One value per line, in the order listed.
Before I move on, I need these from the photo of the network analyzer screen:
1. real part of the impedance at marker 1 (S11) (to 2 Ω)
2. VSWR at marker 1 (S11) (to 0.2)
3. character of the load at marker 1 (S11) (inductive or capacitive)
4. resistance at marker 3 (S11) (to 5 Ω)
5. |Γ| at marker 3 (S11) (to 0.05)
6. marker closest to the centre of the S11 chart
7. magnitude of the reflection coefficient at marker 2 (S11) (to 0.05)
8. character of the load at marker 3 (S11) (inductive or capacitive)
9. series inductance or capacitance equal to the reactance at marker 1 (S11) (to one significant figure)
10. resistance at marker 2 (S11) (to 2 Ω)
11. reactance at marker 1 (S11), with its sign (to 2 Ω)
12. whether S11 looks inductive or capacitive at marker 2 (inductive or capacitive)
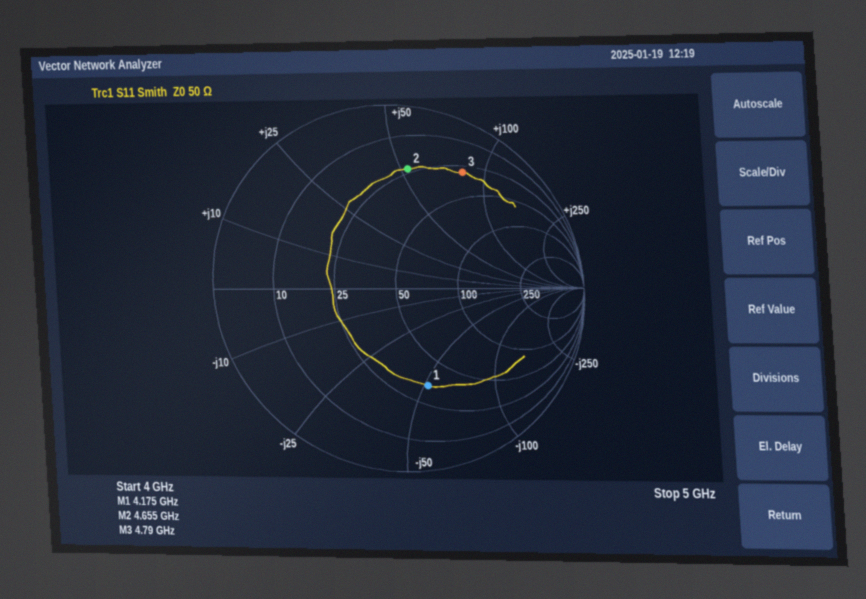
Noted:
34 Ω
3.4
capacitive
30 Ω
0.75
marker 1
0.65
inductive
700 fF
24 Ω
-52 Ω
inductive
